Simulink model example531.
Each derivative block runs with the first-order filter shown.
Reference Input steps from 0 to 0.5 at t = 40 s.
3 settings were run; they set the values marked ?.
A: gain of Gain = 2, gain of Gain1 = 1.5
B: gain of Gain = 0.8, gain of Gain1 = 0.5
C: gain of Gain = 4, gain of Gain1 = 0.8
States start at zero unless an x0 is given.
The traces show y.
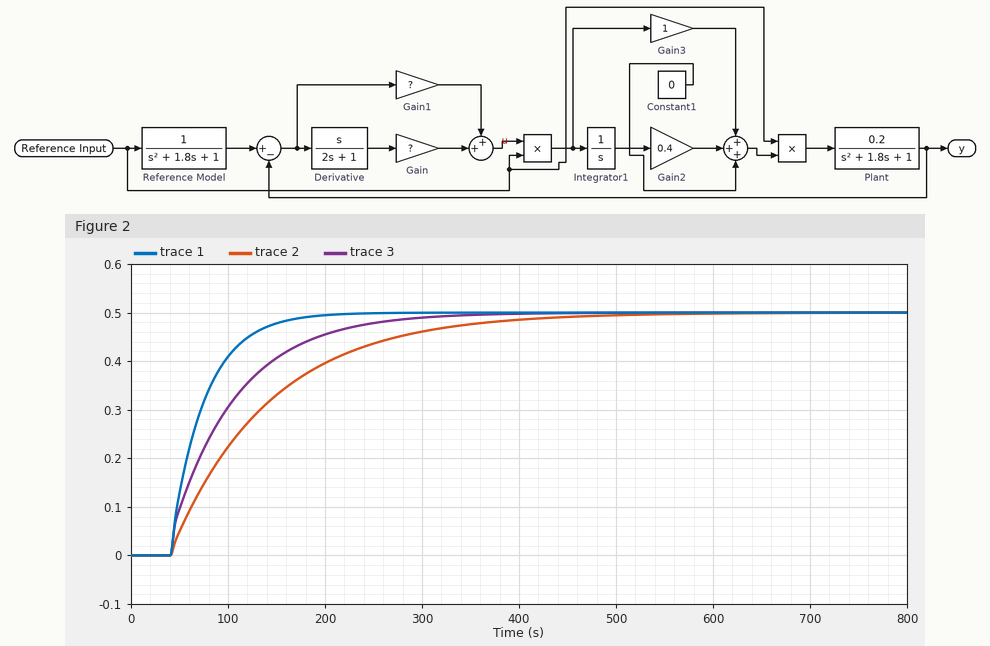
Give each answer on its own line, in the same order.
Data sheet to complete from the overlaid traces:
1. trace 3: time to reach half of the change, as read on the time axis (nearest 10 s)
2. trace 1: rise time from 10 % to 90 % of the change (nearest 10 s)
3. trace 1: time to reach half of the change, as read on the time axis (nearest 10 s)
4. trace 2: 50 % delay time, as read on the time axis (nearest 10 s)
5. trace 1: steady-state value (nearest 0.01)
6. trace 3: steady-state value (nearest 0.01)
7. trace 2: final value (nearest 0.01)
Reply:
80 s
80 s
60 s
110 s
0.50
0.50
0.50
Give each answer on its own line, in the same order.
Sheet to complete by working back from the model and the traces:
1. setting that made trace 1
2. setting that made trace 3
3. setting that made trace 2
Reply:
A
C
B
